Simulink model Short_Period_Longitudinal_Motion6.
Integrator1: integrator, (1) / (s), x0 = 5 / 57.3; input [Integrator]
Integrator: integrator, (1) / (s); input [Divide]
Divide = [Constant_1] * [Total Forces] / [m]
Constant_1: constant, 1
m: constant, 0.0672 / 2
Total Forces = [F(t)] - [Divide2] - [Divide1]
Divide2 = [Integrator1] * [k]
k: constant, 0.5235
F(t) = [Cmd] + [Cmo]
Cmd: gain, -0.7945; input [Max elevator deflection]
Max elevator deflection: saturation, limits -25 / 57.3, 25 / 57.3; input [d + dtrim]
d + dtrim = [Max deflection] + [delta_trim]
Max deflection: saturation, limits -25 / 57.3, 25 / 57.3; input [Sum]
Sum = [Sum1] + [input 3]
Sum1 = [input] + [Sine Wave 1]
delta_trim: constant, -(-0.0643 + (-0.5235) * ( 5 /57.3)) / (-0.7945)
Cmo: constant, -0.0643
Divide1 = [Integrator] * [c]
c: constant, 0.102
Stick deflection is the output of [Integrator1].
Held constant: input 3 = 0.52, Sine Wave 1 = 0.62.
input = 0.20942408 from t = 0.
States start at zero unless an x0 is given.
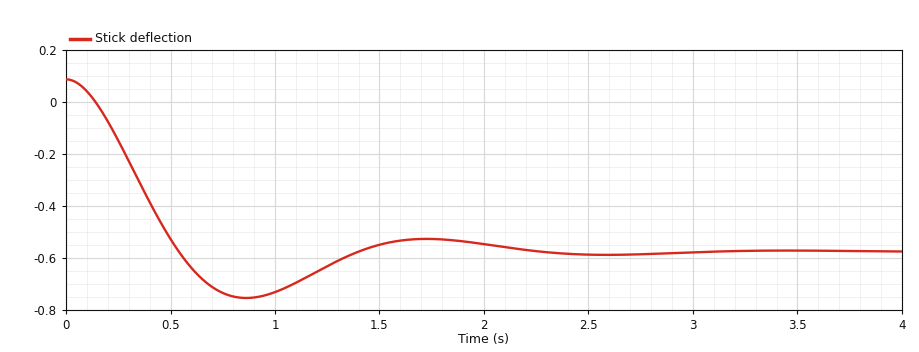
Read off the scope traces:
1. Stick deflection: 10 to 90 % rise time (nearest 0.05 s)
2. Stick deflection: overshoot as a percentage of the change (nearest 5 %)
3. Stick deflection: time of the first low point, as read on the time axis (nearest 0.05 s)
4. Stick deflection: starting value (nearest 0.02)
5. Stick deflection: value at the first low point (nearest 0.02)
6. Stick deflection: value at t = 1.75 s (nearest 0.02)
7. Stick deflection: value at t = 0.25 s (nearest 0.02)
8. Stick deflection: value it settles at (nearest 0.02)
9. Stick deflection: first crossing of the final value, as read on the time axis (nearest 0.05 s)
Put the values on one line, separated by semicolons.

0.35 s; 25 %; 0.85 s; 0.08; -0.76; -0.52; -0.14; -0.58; 0.55 s
